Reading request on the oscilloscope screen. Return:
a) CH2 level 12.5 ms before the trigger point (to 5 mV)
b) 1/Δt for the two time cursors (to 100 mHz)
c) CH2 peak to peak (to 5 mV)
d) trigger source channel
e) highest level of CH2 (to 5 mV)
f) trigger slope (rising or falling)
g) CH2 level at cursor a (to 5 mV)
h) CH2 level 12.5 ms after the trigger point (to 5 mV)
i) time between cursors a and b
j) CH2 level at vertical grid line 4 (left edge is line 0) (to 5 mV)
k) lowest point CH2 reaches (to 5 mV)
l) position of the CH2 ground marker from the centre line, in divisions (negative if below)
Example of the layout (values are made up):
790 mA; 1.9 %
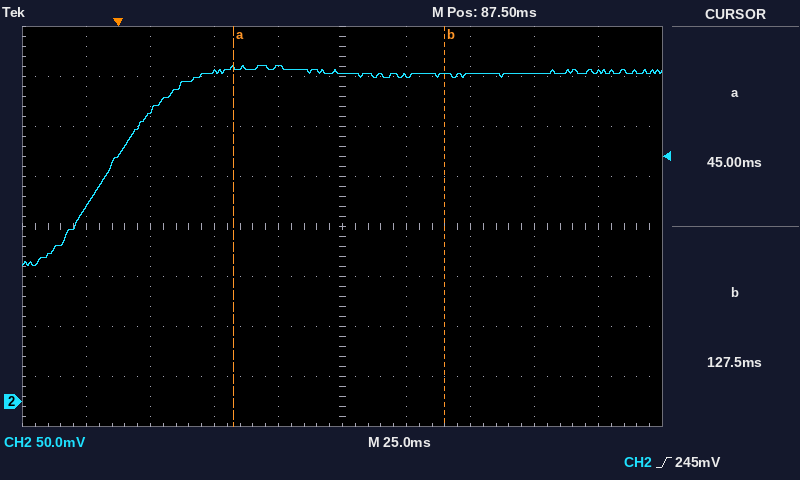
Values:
195 mV; 12.1 Hz; 200 mV; CH2; 335 mV; rising; 335 mV; 290 mV; 82.5 ms; 335 mV; 135 mV; -3.5 div
